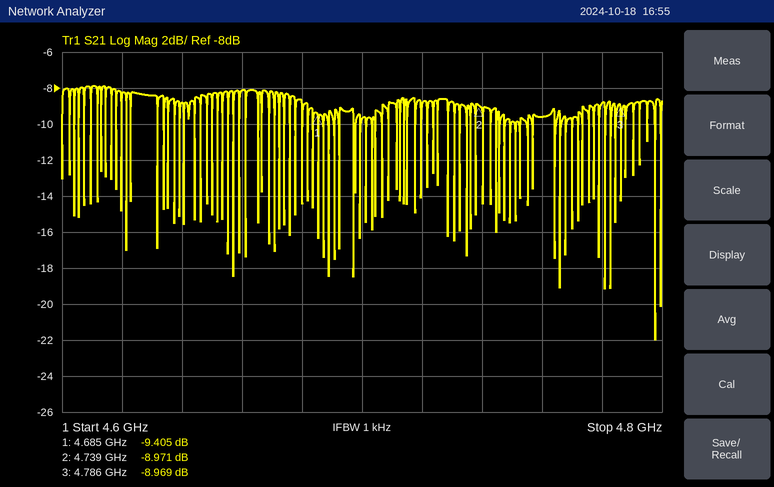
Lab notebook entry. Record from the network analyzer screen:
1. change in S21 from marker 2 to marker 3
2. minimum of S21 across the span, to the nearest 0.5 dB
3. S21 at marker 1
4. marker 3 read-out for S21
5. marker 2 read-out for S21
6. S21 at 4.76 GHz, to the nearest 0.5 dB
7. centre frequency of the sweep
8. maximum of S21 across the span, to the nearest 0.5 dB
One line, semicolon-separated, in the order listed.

0.002 dB; -22.0 dB; -9.405 dB; -8.969 dB; -8.971 dB; -9.5 dB; 4.7 GHz; -8.0 dB
